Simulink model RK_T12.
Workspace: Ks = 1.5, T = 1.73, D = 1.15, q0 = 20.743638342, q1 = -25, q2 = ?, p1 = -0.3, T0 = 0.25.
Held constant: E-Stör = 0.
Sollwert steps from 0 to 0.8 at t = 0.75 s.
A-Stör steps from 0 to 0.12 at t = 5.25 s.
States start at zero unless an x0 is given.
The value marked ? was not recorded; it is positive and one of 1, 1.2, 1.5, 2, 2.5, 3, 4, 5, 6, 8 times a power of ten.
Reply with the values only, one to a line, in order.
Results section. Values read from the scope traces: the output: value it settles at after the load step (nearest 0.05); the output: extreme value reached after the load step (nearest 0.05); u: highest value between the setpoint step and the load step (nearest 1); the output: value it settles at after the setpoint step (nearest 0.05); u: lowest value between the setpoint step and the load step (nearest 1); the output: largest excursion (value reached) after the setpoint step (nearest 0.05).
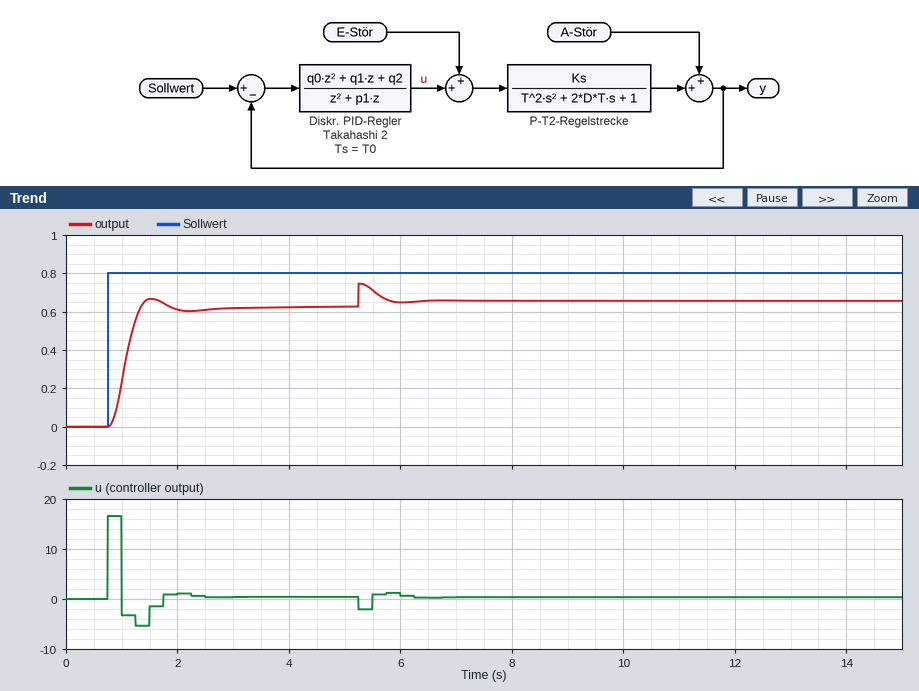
0.65
0.75
17
0.65
-5
0.65
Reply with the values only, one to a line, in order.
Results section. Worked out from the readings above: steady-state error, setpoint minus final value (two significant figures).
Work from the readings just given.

0.15
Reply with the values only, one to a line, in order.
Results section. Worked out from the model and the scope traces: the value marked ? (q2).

6
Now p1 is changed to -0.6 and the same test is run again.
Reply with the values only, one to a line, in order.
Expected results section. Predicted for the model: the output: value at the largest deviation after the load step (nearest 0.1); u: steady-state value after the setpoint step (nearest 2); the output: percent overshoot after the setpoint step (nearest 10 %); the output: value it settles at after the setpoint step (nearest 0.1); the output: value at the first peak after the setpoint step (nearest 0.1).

0.8
0
30 %
0.7
0.9
